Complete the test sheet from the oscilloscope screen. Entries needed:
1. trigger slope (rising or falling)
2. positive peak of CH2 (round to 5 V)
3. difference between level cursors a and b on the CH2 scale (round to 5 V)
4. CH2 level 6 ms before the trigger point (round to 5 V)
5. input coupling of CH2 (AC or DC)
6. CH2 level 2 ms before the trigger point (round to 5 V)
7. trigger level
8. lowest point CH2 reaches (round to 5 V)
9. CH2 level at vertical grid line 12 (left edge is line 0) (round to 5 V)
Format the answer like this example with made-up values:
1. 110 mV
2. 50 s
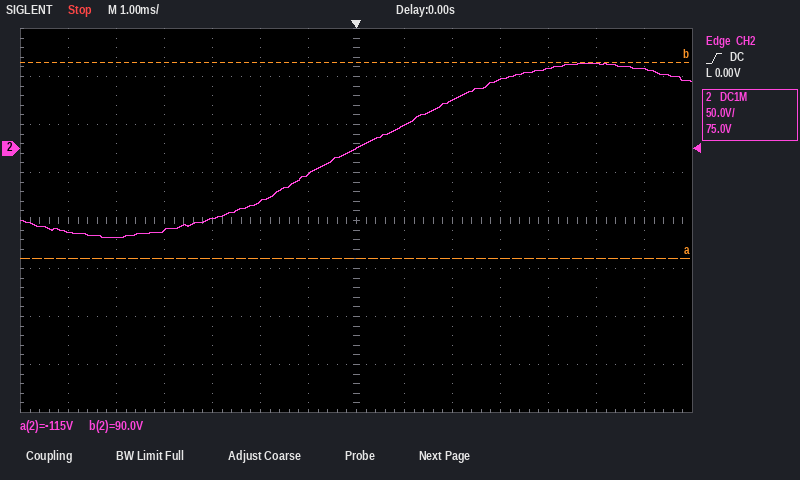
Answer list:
1. rising
2. 90 V
3. 205 V
4. -85 V
5. DC
6. -55 V
7. 0.00 V
8. -95 V
9. 90 V
